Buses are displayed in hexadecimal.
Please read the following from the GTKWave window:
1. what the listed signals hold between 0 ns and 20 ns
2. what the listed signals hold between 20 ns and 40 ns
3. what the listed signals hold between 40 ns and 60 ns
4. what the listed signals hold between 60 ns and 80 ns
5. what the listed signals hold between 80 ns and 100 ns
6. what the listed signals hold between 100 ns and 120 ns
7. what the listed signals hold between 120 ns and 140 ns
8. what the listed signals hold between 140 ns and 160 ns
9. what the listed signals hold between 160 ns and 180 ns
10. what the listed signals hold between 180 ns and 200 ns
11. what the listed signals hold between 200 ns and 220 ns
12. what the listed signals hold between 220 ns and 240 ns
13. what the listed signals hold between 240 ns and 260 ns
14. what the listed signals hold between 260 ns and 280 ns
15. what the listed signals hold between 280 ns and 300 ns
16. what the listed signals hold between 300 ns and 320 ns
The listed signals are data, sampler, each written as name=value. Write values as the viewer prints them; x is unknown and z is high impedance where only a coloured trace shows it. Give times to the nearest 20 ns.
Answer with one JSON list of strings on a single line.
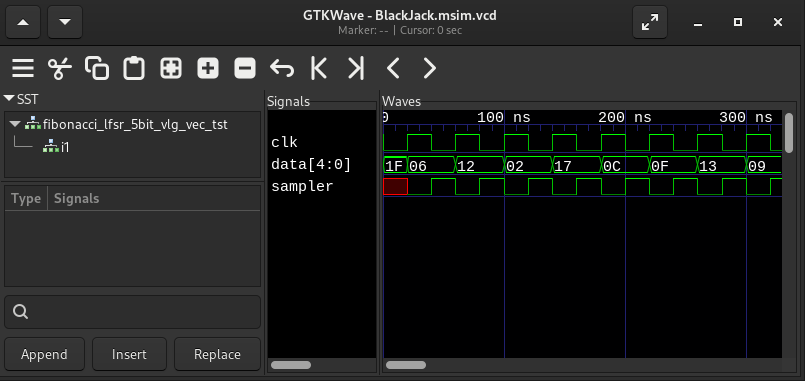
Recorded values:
["data=1F, sampler=x", "data=06, sampler=0", "data=06, sampler=1", "data=12, sampler=0", "data=12, sampler=1", "data=02, sampler=0", "data=02, sampler=1", "data=17, sampler=0", "data=17, sampler=1", "data=0C, sampler=0", "data=0C, sampler=1", "data=0F, sampler=0", "data=0F, sampler=1", "data=13, sampler=0", "data=13, sampler=1", "data=09, sampler=0"]
